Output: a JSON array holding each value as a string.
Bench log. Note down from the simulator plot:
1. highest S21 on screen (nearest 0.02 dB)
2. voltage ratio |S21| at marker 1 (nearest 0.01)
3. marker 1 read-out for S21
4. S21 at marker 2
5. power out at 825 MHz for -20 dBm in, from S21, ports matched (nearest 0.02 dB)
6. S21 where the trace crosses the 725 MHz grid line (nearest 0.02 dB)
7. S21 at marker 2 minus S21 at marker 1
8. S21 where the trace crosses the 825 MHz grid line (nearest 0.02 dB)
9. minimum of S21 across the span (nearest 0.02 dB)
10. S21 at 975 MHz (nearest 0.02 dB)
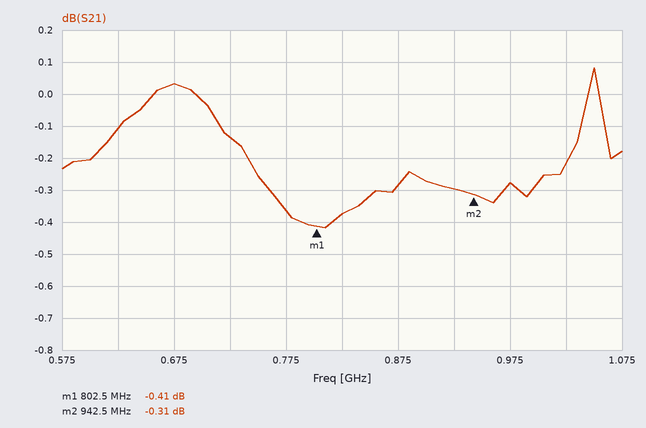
["0.08 dB", "0.95", "-0.41 dB", "-0.31 dB", "-20.38 dBm", "-0.14 dB", "0.10 dB", "-0.38 dB", "-0.42 dB", "-0.28 dB"]
